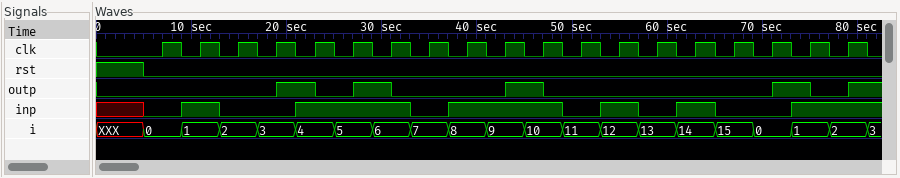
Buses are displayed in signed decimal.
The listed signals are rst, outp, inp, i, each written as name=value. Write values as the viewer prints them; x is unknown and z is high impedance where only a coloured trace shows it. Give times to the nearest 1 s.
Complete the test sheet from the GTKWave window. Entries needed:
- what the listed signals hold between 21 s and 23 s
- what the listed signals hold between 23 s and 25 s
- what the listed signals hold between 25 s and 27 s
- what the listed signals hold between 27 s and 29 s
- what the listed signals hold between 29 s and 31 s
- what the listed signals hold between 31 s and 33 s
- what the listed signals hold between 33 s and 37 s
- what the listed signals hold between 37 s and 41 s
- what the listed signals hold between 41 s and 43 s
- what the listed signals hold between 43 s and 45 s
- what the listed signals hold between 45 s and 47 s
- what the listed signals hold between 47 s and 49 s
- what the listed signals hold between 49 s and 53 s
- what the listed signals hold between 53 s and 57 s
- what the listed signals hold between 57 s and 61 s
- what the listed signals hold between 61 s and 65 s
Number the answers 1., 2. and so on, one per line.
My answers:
1. rst=0, outp=1, inp=1, i=4
2. rst=0, outp=0, inp=1, i=4
3. rst=0, outp=0, inp=1, i=5
4. rst=0, outp=1, inp=1, i=5
5. rst=0, outp=1, inp=1, i=6
6. rst=0, outp=0, inp=1, i=6
7. rst=0, outp=0, inp=0, i=7
8. rst=0, outp=0, inp=1, i=8
9. rst=0, outp=0, inp=1, i=9
10. rst=0, outp=1, inp=1, i=9
11. rst=0, outp=1, inp=1, i=10
12. rst=0, outp=0, inp=1, i=10
13. rst=0, outp=0, inp=0, i=11
14. rst=0, outp=0, inp=1, i=12
15. rst=0, outp=0, inp=0, i=13
16. rst=0, outp=0, inp=1, i=14
